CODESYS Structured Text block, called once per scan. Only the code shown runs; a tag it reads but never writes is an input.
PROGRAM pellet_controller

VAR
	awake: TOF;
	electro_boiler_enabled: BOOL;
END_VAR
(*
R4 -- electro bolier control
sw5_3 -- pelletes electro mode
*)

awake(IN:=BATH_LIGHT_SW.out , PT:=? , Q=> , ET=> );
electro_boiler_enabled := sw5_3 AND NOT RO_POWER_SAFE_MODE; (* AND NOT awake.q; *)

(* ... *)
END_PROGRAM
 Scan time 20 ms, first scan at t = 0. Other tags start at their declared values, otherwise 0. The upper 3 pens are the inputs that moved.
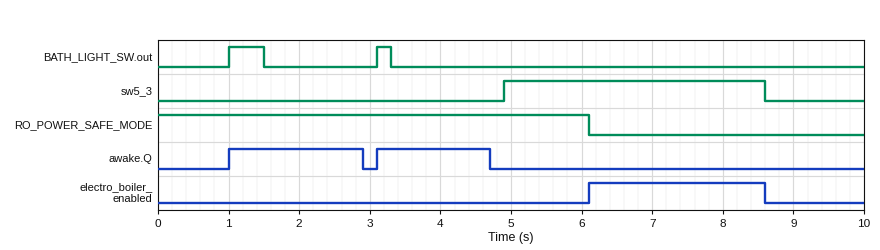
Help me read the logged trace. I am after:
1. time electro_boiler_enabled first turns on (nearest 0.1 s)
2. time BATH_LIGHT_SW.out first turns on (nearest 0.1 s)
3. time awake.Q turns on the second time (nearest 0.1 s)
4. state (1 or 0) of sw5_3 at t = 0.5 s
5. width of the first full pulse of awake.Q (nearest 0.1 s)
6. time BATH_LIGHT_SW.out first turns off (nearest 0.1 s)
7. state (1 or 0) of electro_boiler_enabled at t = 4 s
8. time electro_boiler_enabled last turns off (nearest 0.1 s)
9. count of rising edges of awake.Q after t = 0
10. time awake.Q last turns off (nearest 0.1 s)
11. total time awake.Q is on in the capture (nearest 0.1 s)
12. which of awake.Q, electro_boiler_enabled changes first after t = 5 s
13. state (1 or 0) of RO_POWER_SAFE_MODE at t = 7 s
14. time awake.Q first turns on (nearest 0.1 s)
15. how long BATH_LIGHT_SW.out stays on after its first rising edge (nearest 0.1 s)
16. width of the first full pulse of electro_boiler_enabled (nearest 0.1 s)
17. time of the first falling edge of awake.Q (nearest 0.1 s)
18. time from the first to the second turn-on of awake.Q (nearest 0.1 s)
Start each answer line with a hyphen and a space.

- 6.1 s
- 1.0 s
- 3.1 s
- 0
- 1.9 s
- 1.5 s
- 0
- 8.6 s
- 2
- 4.7 s
- 3.5 s
- electro_boiler_enabled
- 0
- 1.0 s
- 0.5 s
- 2.5 s
- 2.9 s
- 2.1 s
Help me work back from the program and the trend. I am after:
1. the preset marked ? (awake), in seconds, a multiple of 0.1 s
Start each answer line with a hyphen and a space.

- 1.4 s
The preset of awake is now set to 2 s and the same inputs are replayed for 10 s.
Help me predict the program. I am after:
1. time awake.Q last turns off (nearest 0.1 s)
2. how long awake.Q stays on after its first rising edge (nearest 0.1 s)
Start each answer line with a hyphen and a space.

- 5.3 s
- 4.3 s
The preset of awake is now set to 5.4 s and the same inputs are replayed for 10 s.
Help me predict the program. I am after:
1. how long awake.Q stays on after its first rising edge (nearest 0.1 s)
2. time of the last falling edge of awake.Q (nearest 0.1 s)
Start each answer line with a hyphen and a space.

- 7.7 s
- 8.7 s
